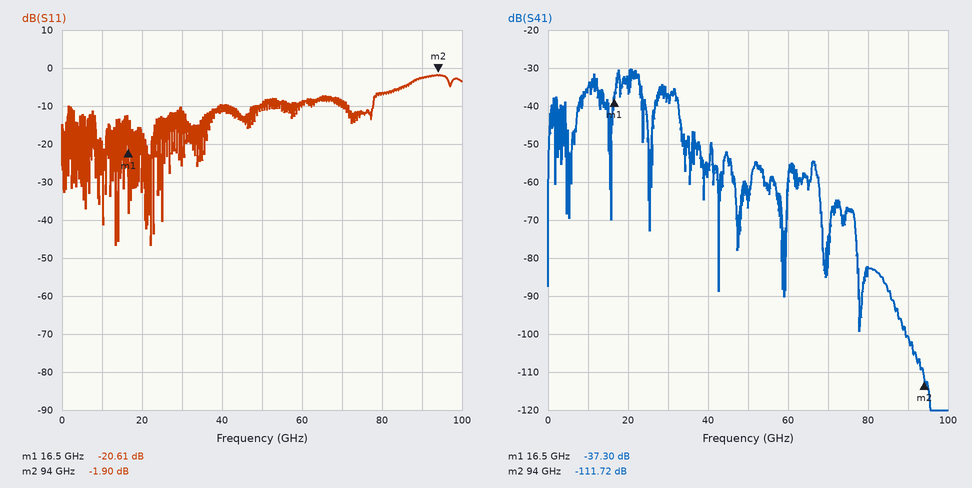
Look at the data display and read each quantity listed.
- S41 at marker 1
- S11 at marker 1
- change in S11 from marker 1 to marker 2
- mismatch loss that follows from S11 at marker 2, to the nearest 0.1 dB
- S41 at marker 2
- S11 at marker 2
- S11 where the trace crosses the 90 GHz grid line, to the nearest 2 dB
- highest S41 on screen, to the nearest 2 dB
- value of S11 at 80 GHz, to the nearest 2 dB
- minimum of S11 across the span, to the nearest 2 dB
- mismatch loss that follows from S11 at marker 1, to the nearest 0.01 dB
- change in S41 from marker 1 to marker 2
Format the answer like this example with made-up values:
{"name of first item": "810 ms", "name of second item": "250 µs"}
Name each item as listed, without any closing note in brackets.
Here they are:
{"S41 at marker 1": "-37.30 dB", "S11 at marker 1": "-20.61 dB", "change in S11 from marker 1 to marker 2": "18.71 dB", "mismatch loss that follows from S11 at marker 2, to the nearest 0.1 dB": "4.5 dB", "S41 at marker 2": "-111.72 dB", "S11 at marker 2": "-1.90 dB", "S11 where the trace crosses the 90 GHz grid line, to the nearest 2 dB": "-2 dB", "highest S41 on screen, to the nearest 2 dB": "-30 dB", "value of S11 at 80 GHz, to the nearest 2 dB": "-6 dB", "minimum of S11 across the span, to the nearest 2 dB": "-46 dB", "mismatch loss that follows from S11 at marker 1, to the nearest 0.01 dB": "0.04 dB", "change in S41 from marker 1 to marker 2": "-74.42 dB"}
